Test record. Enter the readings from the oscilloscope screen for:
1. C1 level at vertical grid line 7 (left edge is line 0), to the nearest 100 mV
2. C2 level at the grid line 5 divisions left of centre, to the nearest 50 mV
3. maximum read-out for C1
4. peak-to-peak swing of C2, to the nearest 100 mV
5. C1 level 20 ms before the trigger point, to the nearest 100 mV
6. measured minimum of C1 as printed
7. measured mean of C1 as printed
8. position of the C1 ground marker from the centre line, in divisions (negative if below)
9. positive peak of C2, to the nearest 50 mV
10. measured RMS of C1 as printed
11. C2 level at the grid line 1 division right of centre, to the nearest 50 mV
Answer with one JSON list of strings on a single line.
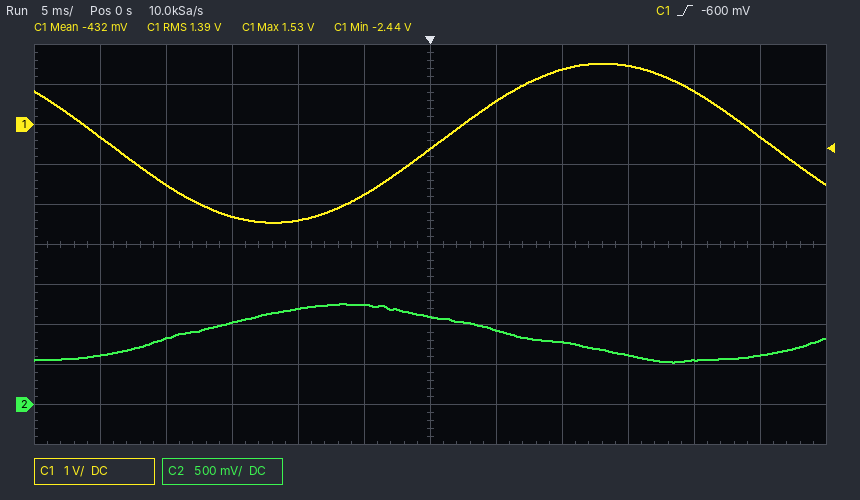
["600 mV", "600 mV", "1.53 V", "700 mV", "-1.5 V", "-2.44 V", "-432 mV", "+3.0 div", "1.25 V", "1.39 V", "950 mV"]
